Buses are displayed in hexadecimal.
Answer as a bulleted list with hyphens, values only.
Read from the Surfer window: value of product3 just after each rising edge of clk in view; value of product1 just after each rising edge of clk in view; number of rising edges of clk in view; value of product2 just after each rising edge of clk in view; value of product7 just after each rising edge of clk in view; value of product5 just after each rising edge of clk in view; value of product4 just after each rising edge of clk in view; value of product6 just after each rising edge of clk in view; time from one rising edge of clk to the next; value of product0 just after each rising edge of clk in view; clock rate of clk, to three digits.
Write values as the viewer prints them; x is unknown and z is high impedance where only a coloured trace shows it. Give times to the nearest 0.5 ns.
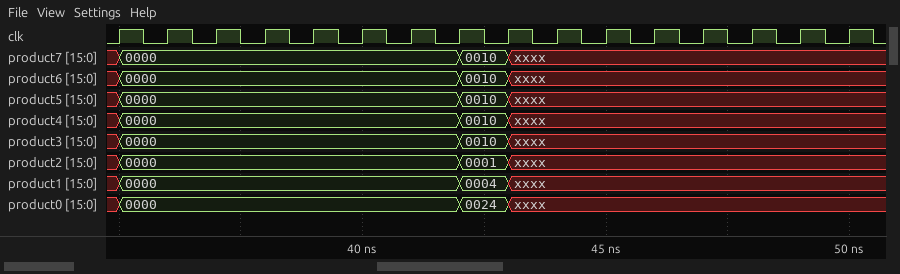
- 0000, 0000, 0000, 0000, 0000, 0000, 0000, 0010, xxxx, xxxx, xxxx, xxxx, xxxx, xxxx, xxxx, xxxx
- 0000, 0000, 0000, 0000, 0000, 0000, 0000, 0004, xxxx, xxxx, xxxx, xxxx, xxxx, xxxx, xxxx, xxxx
- 16
- 0000, 0000, 0000, 0000, 0000, 0000, 0000, 0001, xxxx, xxxx, xxxx, xxxx, xxxx, xxxx, xxxx, xxxx
- 0000, 0000, 0000, 0000, 0000, 0000, 0000, 0010, xxxx, xxxx, xxxx, xxxx, xxxx, xxxx, xxxx, xxxx
- 0000, 0000, 0000, 0000, 0000, 0000, 0000, 0010, xxxx, xxxx, xxxx, xxxx, xxxx, xxxx, xxxx, xxxx
- 0000, 0000, 0000, 0000, 0000, 0000, 0000, 0010, xxxx, xxxx, xxxx, xxxx, xxxx, xxxx, xxxx, xxxx
- 0000, 0000, 0000, 0000, 0000, 0000, 0000, 0010, xxxx, xxxx, xxxx, xxxx, xxxx, xxxx, xxxx, xxxx
- 1 ns
- 0000, 0000, 0000, 0000, 0000, 0000, 0000, 0024, xxxx, xxxx, xxxx, xxxx, xxxx, xxxx, xxxx, xxxx
- 1.00 GHz
